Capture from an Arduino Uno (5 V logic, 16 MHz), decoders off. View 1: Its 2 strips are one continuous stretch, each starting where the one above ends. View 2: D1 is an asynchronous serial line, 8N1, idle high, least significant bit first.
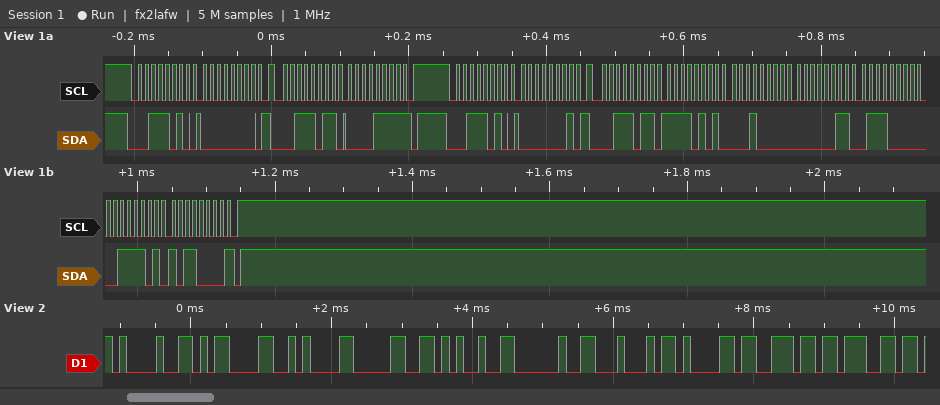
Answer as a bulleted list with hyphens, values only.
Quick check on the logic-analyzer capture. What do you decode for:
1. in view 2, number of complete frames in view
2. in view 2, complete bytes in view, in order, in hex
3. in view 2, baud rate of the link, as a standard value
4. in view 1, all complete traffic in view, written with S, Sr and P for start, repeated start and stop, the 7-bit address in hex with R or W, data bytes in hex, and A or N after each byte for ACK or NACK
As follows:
- 10
- 21 0D 0A 30 25 20 44 61 6E 67
- 9600 baud
- S 1DW A 00 A Sr 1DR A 0F N P S 1DW A 01 A Sr 1DR A F5 A 10 A 03 A 70 A 3D A B0 N P
